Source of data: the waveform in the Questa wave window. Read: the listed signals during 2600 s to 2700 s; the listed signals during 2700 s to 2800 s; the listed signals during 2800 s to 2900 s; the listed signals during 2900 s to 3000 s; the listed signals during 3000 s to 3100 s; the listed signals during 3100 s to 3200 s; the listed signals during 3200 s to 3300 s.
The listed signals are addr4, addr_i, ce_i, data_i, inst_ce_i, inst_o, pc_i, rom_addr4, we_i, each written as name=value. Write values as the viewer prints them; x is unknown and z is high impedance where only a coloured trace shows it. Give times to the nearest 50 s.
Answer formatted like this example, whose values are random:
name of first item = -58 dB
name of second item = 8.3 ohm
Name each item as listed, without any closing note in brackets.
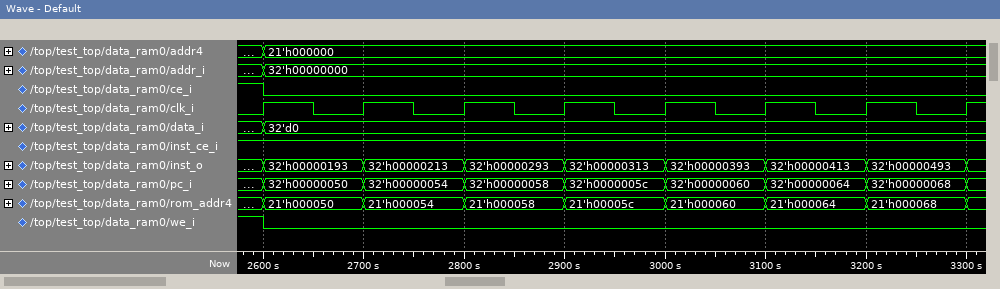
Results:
the listed signals during 2600 s to 2700 s = addr4=21'h000000, addr_i=32'h00000000, ce_i=0, data_i=32'd0, inst_ce_i=1, inst_o=32'h00000193, pc_i=32'h00000050, rom_addr4=21'h000050, we_i=0
the listed signals during 2700 s to 2800 s = addr4=21'h000000, addr_i=32'h00000000, ce_i=0, data_i=32'd0, inst_ce_i=1, inst_o=32'h00000213, pc_i=32'h00000054, rom_addr4=21'h000054, we_i=0
the listed signals during 2800 s to 2900 s = addr4=21'h000000, addr_i=32'h00000000, ce_i=0, data_i=32'd0, inst_ce_i=1, inst_o=32'h00000293, pc_i=32'h00000058, rom_addr4=21'h000058, we_i=0
the listed signals during 2900 s to 3000 s = addr4=21'h000000, addr_i=32'h00000000, ce_i=0, data_i=32'd0, inst_ce_i=1, inst_o=32'h00000313, pc_i=32'h0000005c, rom_addr4=21'h00005c, we_i=0
the listed signals during 3000 s to 3100 s = addr4=21'h000000, addr_i=32'h00000000, ce_i=0, data_i=32'd0, inst_ce_i=1, inst_o=32'h00000393, pc_i=32'h00000060, rom_addr4=21'h000060, we_i=0
the listed signals during 3100 s to 3200 s = addr4=21'h000000, addr_i=32'h00000000, ce_i=0, data_i=32'd0, inst_ce_i=1, inst_o=32'h00000413, pc_i=32'h00000064, rom_addr4=21'h000064, we_i=0
the listed signals during 3200 s to 3300 s = addr4=21'h000000, addr_i=32'h00000000, ce_i=0, data_i=32'd0, inst_ce_i=1, inst_o=32'h00000493, pc_i=32'h00000068, rom_addr4=21'h000068, we_i=0
